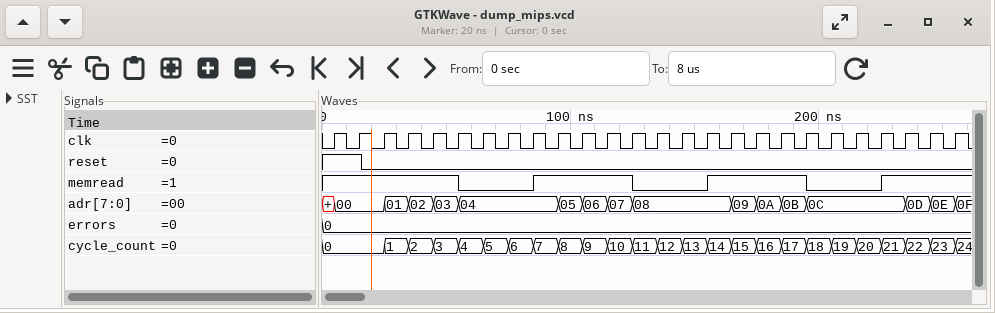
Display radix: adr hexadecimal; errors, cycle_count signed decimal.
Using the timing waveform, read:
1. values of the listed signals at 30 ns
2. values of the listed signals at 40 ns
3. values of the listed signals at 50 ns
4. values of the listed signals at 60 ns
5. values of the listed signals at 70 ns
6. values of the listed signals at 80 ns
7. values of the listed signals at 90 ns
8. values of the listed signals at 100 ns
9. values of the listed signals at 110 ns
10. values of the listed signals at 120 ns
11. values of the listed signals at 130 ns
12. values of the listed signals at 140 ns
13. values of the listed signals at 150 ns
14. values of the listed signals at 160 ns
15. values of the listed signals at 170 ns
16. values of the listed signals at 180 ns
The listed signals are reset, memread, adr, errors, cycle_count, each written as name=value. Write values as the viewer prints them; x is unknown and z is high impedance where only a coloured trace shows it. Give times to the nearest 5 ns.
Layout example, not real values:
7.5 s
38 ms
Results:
reset=0, memread=1, adr=01, errors=0, cycle_count=1
reset=0, memread=1, adr=02, errors=0, cycle_count=2
reset=0, memread=1, adr=03, errors=0, cycle_count=3
reset=0, memread=0, adr=04, errors=0, cycle_count=4
reset=0, memread=0, adr=04, errors=0, cycle_count=5
reset=0, memread=0, adr=04, errors=0, cycle_count=6
reset=0, memread=1, adr=04, errors=0, cycle_count=7
reset=0, memread=1, adr=05, errors=0, cycle_count=8
reset=0, memread=1, adr=06, errors=0, cycle_count=9
reset=0, memread=1, adr=07, errors=0, cycle_count=10
reset=0, memread=0, adr=08, errors=0, cycle_count=11
reset=0, memread=0, adr=08, errors=0, cycle_count=12
reset=0, memread=0, adr=08, errors=0, cycle_count=13
reset=0, memread=1, adr=08, errors=0, cycle_count=14
reset=0, memread=1, adr=09, errors=0, cycle_count=15
reset=0, memread=1, adr=0A, errors=0, cycle_count=16
